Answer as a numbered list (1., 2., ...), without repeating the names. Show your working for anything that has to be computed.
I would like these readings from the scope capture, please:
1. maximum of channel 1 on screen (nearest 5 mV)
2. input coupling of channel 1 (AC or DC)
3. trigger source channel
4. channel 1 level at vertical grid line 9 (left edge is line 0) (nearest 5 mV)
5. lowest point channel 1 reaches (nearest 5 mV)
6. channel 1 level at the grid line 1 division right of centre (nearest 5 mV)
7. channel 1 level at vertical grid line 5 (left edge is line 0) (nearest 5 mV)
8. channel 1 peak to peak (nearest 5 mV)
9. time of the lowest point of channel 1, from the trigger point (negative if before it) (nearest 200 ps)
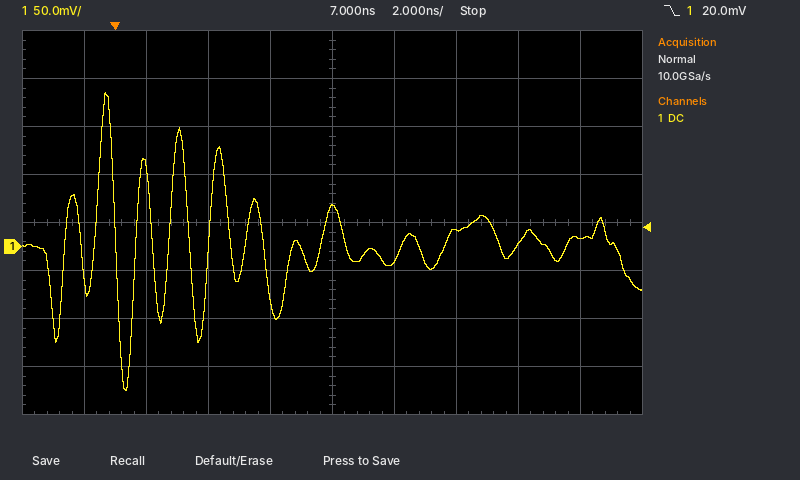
1. 160 mV
2. DC
3. channel 1
4. 10 mV
5. -150 mV
6. -15 mV
7. 40 mV
8. 160 mV − (-150 mV) = 310 mV
9. +400 ps
